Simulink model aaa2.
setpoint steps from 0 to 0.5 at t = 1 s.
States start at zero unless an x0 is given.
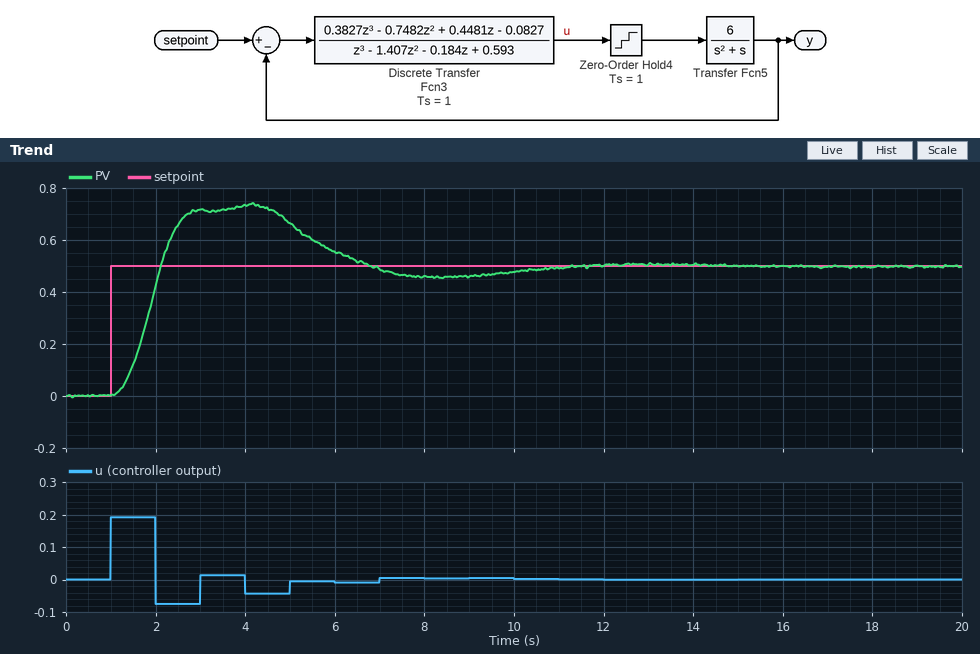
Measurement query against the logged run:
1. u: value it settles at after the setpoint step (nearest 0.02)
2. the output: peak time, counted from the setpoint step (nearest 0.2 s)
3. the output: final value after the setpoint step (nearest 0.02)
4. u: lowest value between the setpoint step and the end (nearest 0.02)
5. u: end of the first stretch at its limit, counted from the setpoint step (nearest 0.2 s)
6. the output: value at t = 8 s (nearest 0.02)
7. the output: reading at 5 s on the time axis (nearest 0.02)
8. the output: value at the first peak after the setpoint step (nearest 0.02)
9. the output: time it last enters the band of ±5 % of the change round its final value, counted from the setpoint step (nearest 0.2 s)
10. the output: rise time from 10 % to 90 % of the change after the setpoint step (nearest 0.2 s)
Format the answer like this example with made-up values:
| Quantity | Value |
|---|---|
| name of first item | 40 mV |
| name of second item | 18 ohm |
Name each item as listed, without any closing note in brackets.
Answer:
| Quantity | Value |
|---|---|
| u: value it settles at after the setpoint step | 0.00 |
| the output: peak time, counted from the setpoint step | 3.2 s |
| the output: final value after the setpoint step | 0.50 |
| u: lowest value between the setpoint step and the end | -0.08 |
| u: end of the first stretch at its limit, counted from the setpoint step | 1.0 s |
| the output: value at t = 8 s | 0.46 |
| the output: reading at 5 s on the time axis | 0.66 |
| the output: value at the first peak after the setpoint step | 0.74 |
| the output: time it last enters the band of ±5 % of the change round its final value, counted from the setpoint step | 8.8 s |
| the output: rise time from 10 % to 90 % of the change after the setpoint step | 0.8 s |
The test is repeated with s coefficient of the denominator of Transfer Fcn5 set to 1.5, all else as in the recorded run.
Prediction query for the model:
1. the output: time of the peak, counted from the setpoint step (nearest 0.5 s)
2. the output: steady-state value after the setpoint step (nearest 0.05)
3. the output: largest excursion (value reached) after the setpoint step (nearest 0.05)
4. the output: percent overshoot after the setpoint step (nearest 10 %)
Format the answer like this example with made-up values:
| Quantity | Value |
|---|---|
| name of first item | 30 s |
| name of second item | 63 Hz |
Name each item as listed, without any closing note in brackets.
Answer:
| Quantity | Value |
|---|---|
| the output: time of the peak, counted from the setpoint step | 3.5 s |
| the output: steady-state value after the setpoint step | 0.50 |
| the output: largest excursion (value reached) after the setpoint step | 0.70 |
| the output: percent overshoot after the setpoint step | 40 % |
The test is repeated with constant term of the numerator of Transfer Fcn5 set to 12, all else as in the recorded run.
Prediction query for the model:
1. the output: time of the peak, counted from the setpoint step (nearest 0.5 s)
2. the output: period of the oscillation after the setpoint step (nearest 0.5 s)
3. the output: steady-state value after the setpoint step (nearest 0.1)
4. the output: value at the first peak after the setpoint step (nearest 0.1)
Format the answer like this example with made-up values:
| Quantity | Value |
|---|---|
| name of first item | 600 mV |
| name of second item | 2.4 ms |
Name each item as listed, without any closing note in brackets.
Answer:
| Quantity | Value |
|---|---|
| the output: time of the peak, counted from the setpoint step | 1.5 s |
| the output: period of the oscillation after the setpoint step | 3.0 s |
| the output: steady-state value after the setpoint step | 0.5 |
| the output: value at the first peak after the setpoint step | 1.1 |
